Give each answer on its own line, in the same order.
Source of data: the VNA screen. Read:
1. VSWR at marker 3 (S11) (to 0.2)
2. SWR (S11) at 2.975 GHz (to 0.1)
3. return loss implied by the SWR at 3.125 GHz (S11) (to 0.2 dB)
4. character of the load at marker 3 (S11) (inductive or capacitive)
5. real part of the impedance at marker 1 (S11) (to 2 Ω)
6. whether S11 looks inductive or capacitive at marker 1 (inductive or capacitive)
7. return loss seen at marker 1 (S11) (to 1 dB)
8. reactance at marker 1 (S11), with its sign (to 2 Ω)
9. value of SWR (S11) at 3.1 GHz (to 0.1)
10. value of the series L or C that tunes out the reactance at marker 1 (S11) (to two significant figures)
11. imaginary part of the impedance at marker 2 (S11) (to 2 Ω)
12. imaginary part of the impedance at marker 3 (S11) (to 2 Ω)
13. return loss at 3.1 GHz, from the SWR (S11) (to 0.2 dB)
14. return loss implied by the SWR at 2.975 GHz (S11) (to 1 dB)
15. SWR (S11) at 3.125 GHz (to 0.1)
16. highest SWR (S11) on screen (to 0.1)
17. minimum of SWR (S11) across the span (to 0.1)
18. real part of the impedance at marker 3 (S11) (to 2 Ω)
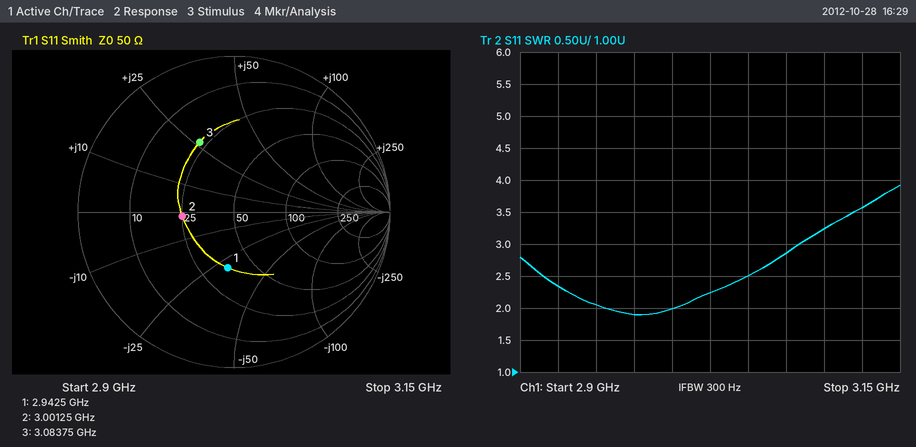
3.0
1.9
5.0 dB
inductive
36 Ω
capacitive
9 dB
-30 Ω
3.2
1.6 nH
-2 Ω
+26 Ω
5.6 dB
10 dB
3.6
3.9
1.9
22 Ω
